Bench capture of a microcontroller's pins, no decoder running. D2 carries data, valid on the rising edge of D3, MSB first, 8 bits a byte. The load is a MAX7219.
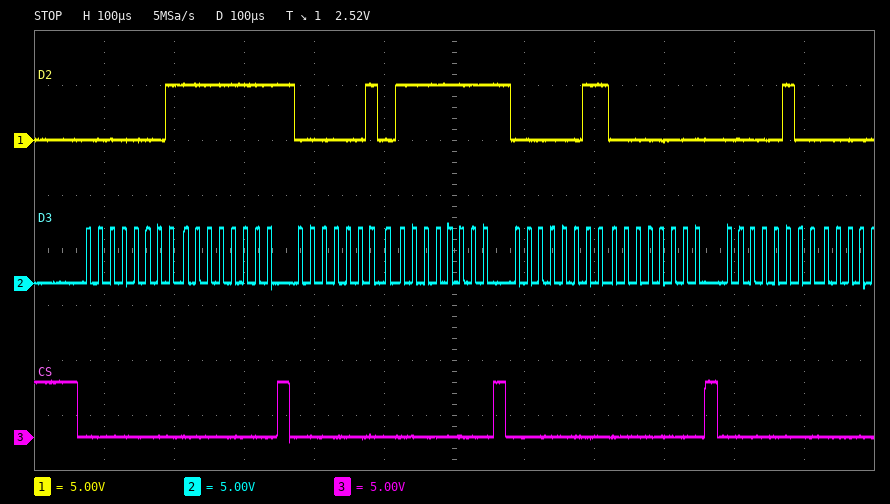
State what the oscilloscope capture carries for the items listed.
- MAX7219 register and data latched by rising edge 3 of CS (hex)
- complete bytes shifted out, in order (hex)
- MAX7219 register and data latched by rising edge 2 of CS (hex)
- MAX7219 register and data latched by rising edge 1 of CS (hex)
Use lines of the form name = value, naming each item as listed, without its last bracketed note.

MAX7219 register and data latched by rising edge 3 of CS = register 0x3, data 0x00
complete bytes shifted out, in order = 0x01 0xFF 0x02 0xFF 0x03 0x00 0x04
MAX7219 register and data latched by rising edge 2 of CS = register 0x2, data 0xFF
MAX7219 register and data latched by rising edge 1 of CS = register 0x1, data 0xFF
